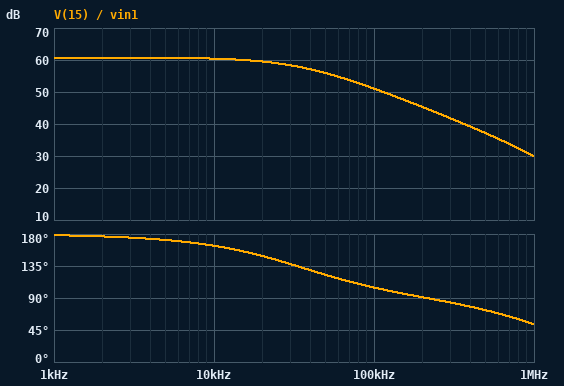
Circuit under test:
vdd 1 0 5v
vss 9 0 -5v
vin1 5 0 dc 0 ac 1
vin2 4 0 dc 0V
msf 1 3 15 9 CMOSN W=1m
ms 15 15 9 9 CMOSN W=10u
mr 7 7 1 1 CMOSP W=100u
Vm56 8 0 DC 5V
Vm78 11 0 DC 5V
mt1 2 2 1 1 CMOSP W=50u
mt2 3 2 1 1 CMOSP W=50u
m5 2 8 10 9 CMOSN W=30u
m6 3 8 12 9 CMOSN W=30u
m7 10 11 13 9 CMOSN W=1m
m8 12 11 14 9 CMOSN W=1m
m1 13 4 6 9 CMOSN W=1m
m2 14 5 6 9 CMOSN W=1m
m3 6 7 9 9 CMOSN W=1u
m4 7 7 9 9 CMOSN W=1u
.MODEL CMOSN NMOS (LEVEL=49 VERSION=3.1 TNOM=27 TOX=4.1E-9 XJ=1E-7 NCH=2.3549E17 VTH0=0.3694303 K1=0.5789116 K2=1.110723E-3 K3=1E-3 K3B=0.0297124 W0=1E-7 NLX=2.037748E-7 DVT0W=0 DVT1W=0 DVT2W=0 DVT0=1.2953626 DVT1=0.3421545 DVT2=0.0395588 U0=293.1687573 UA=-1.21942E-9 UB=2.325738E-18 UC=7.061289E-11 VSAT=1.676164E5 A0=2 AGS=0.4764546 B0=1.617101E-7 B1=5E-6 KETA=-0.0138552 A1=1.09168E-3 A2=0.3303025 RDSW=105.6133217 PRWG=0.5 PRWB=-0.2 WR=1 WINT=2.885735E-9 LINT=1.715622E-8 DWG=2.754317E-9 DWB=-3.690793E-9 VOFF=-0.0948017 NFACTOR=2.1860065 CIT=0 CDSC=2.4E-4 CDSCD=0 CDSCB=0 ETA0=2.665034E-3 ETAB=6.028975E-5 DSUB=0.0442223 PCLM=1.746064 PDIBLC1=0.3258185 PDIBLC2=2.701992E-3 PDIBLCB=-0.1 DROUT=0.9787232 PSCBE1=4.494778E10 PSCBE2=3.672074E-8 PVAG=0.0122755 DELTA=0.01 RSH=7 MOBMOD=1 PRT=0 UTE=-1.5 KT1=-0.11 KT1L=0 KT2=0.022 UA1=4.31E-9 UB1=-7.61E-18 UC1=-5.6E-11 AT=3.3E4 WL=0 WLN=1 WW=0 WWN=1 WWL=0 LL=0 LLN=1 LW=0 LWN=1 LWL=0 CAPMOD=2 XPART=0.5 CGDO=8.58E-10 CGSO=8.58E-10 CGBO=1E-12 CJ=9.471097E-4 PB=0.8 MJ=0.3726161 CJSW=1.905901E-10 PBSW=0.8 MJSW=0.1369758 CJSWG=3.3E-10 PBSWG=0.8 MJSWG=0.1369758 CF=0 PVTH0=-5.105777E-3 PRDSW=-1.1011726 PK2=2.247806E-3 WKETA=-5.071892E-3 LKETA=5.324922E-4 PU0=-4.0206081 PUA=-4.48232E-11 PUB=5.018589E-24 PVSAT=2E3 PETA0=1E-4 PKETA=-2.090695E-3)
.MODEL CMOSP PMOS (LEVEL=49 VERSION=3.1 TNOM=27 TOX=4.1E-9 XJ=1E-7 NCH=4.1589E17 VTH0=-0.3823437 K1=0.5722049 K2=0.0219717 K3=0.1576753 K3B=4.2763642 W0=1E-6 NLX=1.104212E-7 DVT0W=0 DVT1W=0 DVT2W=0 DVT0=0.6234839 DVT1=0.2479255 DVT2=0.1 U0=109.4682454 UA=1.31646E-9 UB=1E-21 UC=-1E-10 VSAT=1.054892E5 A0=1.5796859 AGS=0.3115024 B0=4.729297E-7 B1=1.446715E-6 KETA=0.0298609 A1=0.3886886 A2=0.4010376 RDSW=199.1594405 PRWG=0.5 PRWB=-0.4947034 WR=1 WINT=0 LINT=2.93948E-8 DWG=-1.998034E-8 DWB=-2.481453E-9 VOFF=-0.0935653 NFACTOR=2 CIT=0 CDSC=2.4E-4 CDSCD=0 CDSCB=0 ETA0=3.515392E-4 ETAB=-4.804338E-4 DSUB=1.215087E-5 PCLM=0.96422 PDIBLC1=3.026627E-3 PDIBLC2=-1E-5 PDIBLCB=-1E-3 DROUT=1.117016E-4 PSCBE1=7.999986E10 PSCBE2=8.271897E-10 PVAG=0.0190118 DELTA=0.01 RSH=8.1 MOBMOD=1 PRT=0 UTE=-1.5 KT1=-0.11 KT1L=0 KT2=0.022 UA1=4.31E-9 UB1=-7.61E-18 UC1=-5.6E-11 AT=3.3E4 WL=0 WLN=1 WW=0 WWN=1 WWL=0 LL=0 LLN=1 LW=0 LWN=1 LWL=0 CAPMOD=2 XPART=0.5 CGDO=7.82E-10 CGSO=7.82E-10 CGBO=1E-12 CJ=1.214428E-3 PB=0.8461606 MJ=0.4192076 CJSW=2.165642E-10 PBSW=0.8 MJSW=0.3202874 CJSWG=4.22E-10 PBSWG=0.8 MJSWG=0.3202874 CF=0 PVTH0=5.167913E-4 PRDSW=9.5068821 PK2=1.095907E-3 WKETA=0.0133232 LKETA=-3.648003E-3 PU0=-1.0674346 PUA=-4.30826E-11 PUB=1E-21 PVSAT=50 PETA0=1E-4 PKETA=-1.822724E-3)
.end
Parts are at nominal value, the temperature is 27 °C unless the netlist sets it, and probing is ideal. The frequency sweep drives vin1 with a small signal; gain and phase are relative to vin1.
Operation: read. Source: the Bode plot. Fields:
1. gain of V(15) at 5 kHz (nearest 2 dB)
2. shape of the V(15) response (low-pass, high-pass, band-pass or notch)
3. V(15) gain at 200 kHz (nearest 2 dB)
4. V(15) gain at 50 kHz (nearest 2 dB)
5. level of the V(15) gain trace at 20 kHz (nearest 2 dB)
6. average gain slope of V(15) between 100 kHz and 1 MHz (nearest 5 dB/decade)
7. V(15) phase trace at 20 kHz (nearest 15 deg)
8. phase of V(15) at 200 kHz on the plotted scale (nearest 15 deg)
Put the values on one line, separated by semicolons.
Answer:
60 dB; low-pass; 46 dB; 56 dB; 60 dB; -20 dB/decade; 150 deg; 90 deg
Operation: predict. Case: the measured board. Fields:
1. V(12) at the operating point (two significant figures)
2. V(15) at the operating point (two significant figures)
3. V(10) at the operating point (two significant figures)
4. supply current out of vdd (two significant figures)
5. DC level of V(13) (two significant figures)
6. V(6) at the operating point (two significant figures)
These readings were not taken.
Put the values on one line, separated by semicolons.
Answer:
3.1 V; 2.2 V; 3.1 V; 3.8 mA; 3.1 V; -1.1 V
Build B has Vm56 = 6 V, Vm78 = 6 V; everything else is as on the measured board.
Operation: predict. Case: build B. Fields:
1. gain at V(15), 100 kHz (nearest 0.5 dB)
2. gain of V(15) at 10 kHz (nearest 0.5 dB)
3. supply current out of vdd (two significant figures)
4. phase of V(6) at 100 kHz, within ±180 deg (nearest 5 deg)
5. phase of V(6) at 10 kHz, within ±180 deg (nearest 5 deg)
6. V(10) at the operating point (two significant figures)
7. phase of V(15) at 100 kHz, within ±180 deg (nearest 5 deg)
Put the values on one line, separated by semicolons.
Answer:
35.5 dB; 51.5 dB; 3.8 mA; 5 deg; 25 deg; 3.9 V; 95 deg
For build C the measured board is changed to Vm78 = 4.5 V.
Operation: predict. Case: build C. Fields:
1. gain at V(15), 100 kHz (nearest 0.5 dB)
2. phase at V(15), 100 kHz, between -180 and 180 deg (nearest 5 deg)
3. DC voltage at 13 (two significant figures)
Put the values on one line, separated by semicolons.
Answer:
51.5 dB; 110 deg; 2.9 V
